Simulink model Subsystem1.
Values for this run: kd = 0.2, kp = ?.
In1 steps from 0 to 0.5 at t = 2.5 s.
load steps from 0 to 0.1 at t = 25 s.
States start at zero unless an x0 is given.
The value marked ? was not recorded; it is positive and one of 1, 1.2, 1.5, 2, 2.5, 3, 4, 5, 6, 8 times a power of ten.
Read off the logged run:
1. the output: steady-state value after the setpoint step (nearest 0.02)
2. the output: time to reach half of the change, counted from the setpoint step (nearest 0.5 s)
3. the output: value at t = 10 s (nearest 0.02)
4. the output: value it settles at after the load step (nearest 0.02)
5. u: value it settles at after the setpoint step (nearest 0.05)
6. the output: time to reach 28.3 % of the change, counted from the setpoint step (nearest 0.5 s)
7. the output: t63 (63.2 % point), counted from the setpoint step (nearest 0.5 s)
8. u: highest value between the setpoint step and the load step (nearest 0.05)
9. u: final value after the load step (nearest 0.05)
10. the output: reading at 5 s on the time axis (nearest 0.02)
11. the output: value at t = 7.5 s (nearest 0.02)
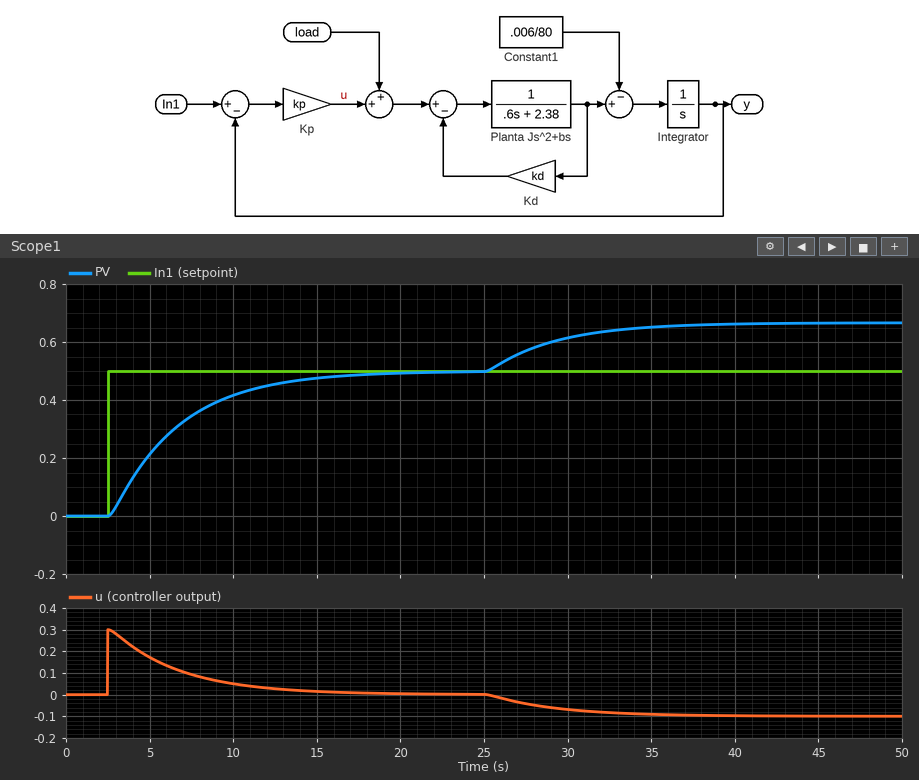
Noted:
0.50
3.0 s
0.42
0.66
0.00
1.5 s
4.5 s
0.30
-0.10
0.22
0.34
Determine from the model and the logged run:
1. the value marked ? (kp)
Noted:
0.6
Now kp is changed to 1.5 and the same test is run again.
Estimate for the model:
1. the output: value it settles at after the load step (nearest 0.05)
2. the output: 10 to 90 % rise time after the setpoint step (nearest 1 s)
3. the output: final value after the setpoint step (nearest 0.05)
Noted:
0.55
3 s
0.50
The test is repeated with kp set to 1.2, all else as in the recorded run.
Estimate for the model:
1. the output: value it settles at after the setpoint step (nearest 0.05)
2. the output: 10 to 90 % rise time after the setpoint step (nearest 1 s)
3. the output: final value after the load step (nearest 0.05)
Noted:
0.50
4 s
0.60
